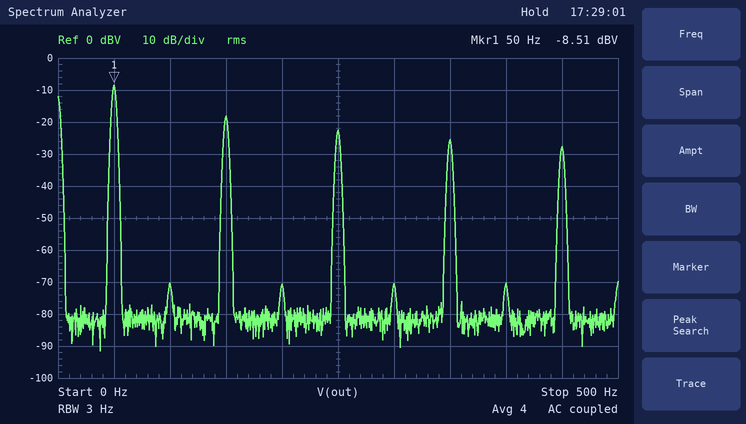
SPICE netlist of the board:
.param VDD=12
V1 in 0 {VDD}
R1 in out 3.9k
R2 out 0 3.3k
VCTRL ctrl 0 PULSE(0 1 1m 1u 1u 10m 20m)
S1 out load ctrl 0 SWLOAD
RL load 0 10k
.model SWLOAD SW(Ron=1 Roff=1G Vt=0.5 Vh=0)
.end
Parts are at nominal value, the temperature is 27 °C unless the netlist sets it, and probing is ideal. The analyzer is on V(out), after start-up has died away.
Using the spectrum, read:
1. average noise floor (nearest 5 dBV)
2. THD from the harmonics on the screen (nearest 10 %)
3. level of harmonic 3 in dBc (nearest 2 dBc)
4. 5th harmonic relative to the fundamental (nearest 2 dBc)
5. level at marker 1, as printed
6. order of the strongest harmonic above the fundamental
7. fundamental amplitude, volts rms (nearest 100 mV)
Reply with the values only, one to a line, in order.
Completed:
-80 dBV
40 %
-10 dBc
-14 dBc
-8.51 dBV
3
400 mV
